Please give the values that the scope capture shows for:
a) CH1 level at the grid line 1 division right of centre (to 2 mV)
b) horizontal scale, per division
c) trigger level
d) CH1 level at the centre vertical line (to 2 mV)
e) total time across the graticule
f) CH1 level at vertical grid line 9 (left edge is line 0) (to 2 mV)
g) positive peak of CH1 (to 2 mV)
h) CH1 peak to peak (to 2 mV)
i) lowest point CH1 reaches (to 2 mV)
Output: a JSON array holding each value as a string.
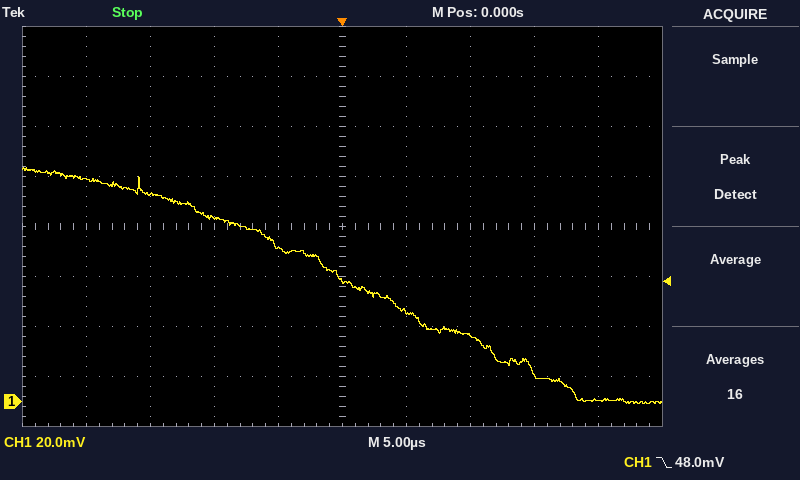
["36 mV", "5 µs", "48.0 mV", "48 mV", "50 µs", "0 mV", "94 mV", "94 mV", "0 mV"]
